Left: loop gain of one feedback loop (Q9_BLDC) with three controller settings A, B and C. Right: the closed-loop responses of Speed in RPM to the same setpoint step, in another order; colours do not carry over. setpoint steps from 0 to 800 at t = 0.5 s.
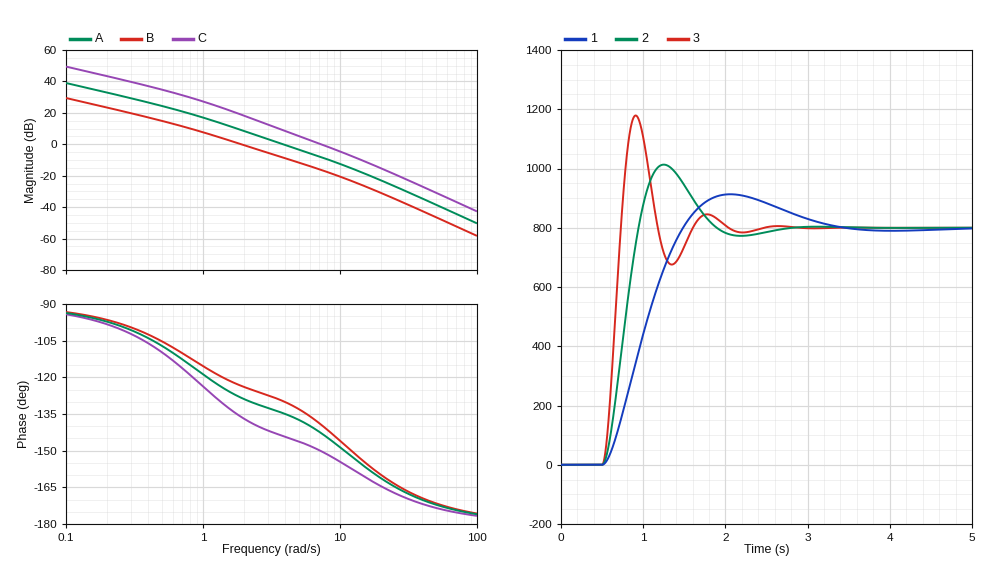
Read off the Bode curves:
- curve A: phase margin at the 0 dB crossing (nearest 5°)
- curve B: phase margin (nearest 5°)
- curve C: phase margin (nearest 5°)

45°
55°
30°
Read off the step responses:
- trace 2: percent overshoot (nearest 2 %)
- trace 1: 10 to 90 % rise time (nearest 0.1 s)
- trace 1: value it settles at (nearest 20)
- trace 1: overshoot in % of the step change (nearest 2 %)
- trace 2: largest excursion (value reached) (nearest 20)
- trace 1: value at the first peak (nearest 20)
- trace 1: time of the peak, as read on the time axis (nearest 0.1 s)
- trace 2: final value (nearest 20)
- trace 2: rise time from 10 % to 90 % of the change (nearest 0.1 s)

26 %
0.7 s
800
14 %
1020
920
2.1 s
800
0.3 s
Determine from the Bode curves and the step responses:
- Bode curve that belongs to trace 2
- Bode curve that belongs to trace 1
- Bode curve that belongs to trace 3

A
B
C
